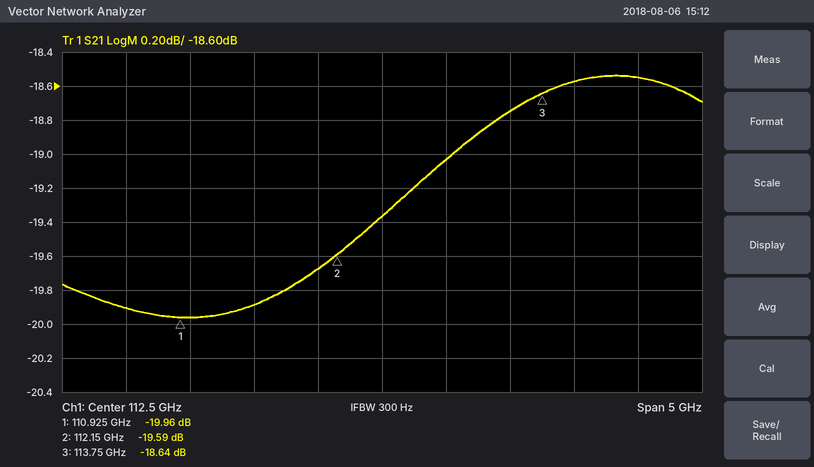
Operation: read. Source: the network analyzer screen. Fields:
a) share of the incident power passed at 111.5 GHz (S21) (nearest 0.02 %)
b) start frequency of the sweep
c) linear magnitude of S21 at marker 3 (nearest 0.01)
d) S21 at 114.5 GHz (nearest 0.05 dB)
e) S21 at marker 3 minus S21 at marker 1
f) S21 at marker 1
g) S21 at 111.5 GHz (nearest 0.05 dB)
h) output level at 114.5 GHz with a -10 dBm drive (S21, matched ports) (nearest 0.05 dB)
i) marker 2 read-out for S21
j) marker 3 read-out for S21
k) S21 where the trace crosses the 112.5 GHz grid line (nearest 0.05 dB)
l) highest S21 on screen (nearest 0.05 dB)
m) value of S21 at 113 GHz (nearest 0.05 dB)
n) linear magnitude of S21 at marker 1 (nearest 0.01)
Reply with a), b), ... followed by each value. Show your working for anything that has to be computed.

a) 10^(-19.9/10) ≈ 1.02 %
b) 110 GHz
c) 10^(-18.64/20) ≈ 0.12
d) -18.55 dB
e) -18.64 − (-19.96) = 1.32 dB
f) -19.96 dB
g) -19.90 dB
h) -10 dBm + (-18.55 dB) = -28.55 dBm
i) -19.59 dB
j) -18.64 dB
k) -19.35 dB
l) -18.55 dB
m) -19.05 dB
n) 10^(-19.96/20) ≈ 0.10
